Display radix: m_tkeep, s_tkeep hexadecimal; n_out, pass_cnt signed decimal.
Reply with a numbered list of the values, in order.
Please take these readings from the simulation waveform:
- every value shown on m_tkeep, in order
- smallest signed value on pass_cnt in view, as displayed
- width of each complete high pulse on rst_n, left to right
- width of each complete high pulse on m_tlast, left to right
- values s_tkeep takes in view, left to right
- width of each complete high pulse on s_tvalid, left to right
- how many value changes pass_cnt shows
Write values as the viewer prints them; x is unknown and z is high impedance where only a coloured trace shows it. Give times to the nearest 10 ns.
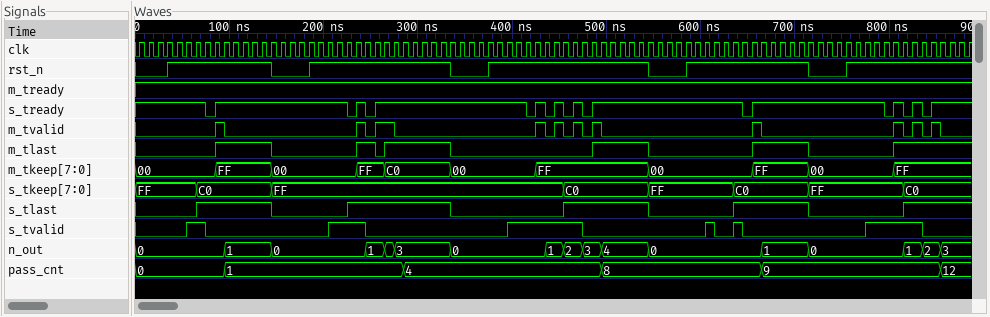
1. 00, FF, 00, FF, C0, 00, FF, 00, FF, 00, FF
2. 0
3. 110 ns, 150 ns, 170 ns, 130 ns
4. 60 ns, 20 ns, 70 ns, 60 ns, 60 ns
5. FF, C0, FF, C0, FF, C0, FF, C0
6. 20 ns, 40 ns, 80 ns, 10 ns, 10 ns, 60 ns
7. 5
